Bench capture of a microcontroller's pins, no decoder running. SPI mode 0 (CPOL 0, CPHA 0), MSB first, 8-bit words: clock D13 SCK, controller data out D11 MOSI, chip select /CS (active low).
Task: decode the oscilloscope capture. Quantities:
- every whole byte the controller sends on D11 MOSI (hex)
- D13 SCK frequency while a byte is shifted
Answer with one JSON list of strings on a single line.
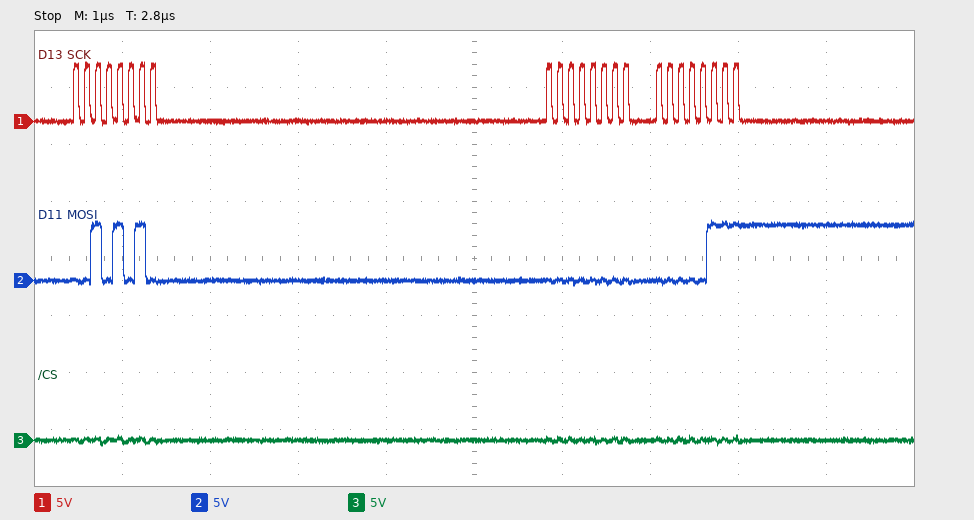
["2A 00 07", "8 MHz"]
